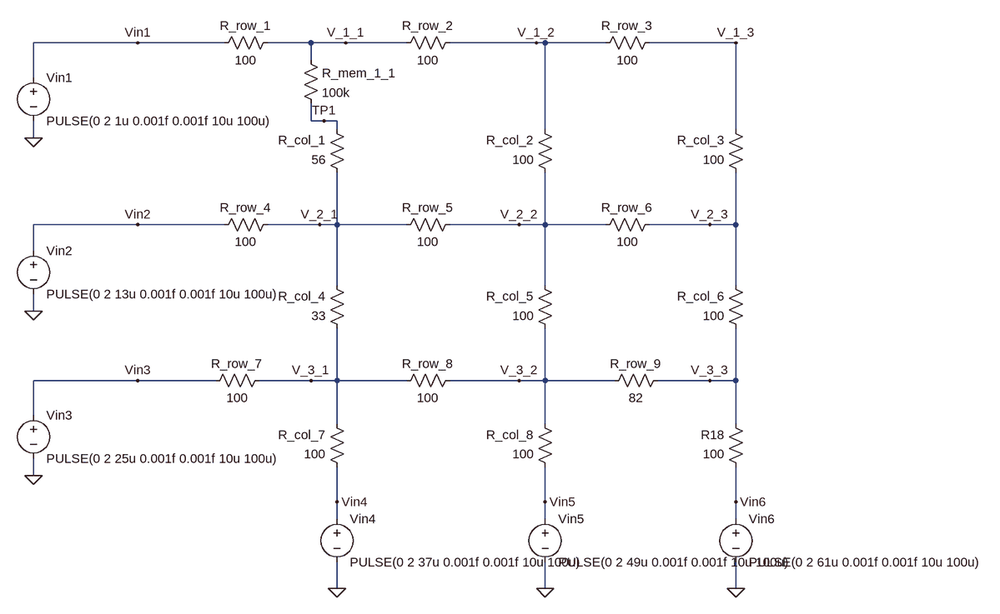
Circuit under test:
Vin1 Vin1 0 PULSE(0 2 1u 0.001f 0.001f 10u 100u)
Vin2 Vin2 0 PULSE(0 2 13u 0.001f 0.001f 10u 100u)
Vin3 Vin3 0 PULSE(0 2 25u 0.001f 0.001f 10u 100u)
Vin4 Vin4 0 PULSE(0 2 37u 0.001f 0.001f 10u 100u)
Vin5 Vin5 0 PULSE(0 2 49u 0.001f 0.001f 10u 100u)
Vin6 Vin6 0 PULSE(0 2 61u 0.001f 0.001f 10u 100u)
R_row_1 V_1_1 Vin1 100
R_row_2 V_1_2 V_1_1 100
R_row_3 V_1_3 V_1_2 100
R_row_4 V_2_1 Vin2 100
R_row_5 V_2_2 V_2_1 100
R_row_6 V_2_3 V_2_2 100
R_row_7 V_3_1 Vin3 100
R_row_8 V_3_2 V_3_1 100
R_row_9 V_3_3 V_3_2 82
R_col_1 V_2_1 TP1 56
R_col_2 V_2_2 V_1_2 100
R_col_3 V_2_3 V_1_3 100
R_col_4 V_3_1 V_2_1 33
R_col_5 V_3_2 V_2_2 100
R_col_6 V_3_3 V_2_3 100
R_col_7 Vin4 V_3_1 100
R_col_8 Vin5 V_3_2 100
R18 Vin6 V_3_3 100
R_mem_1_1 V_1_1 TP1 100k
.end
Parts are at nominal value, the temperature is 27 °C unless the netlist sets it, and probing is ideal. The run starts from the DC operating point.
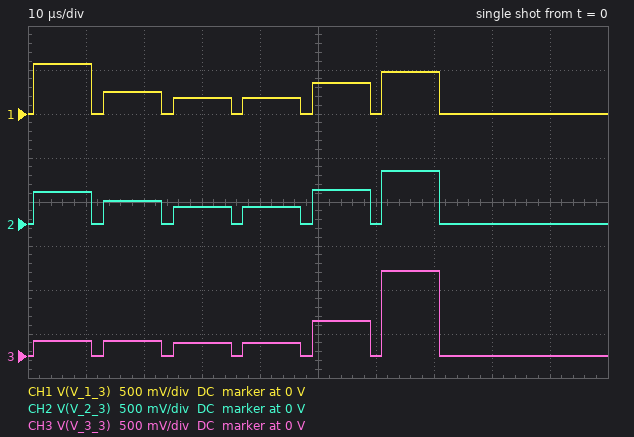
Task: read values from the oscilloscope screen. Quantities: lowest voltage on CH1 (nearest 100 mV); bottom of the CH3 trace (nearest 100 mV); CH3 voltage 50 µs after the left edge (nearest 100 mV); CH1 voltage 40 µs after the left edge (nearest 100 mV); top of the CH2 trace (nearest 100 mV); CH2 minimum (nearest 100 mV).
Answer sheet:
0 V
0 V
400 mV
200 mV
600 mV
0 V
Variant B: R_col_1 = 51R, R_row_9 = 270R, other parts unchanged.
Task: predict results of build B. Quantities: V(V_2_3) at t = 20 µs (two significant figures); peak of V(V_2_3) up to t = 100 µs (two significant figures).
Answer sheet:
250 mV
690 mV
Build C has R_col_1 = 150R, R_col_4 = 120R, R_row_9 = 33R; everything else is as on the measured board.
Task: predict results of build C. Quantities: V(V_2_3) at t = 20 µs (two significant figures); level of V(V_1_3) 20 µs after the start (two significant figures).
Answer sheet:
310 mV
300 mV
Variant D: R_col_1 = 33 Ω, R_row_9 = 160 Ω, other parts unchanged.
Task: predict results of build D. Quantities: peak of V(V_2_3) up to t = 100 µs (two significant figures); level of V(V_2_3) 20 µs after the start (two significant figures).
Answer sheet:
650 mV
250 mV
